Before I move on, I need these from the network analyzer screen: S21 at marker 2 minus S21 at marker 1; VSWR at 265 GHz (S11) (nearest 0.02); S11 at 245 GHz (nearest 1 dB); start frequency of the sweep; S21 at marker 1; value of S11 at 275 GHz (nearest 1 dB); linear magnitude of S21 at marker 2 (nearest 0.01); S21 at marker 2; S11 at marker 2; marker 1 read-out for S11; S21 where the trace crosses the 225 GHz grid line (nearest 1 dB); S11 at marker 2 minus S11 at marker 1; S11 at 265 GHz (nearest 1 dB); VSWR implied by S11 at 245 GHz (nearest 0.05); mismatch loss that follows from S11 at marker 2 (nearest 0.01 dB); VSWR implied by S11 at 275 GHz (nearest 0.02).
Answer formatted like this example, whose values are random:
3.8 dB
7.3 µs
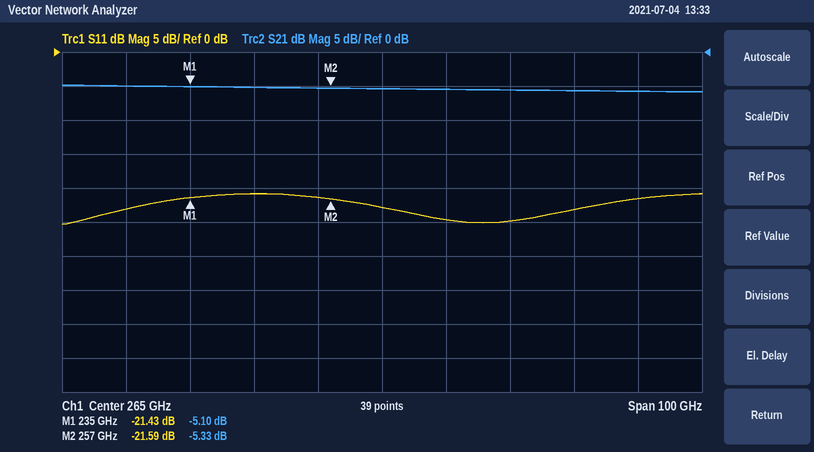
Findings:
-0.23 dB
1.16
-21 dB
215 GHz
-5.10 dB
-25 dB
0.54
-5.33 dB
-21.59 dB
-21.43 dB
-5 dB
-0.16 dB
-23 dB
1.20
0.03 dB
1.12
